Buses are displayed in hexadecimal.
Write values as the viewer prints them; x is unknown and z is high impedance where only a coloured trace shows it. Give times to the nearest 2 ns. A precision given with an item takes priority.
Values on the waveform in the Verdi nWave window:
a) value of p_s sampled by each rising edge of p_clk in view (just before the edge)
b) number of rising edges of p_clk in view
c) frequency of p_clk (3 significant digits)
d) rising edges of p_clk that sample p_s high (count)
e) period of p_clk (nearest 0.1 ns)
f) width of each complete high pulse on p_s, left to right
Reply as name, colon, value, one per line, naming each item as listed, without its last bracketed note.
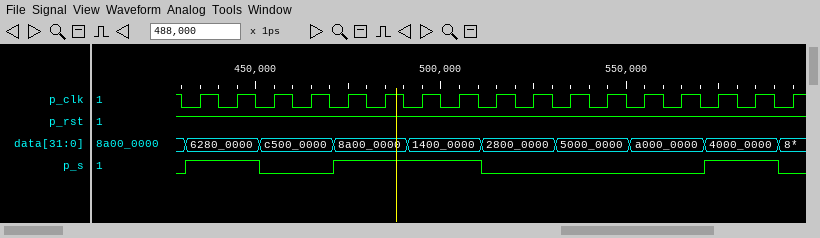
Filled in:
value of p_s sampled by each rising edge of p_clk in view: 1 1 0 0 1 1 1 1 0 0 0 0 0 0 1 1 0
number of rising edges of p_clk in view: 17
frequency of p_clk: 100 MHz
rising edges of p_clk that sample p_s high: 8
period of p_clk: 10 ns
width of each complete high pulse on p_s, left to right: 20 ns, 40 ns, 20 ns
